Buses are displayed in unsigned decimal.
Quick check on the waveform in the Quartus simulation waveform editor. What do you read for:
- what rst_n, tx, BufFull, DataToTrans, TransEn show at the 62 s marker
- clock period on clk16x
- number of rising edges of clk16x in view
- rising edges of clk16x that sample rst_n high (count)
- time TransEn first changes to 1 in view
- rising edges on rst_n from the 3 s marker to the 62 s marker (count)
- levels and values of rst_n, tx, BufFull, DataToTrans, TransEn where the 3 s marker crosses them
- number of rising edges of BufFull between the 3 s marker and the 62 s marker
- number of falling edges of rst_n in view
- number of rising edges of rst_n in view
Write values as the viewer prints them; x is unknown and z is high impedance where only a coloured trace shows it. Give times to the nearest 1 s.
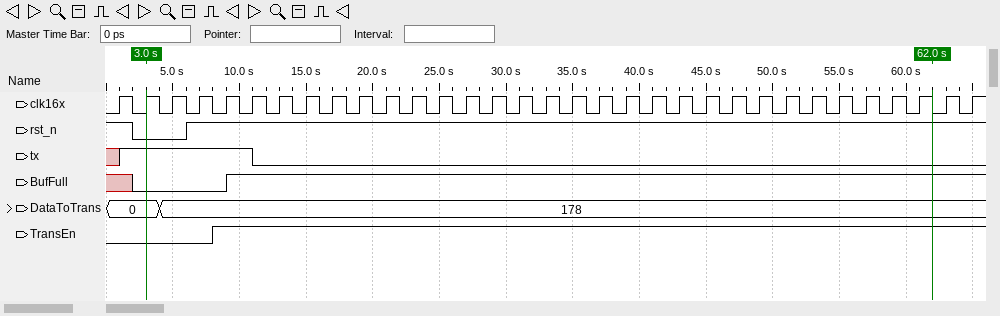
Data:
rst_n=1, tx=0, BufFull=1, DataToTrans=178, TransEn=1
2 s
33
31
8 s
1
rst_n=0, tx=1, BufFull=0, DataToTrans=0, TransEn=0
1
1
1
